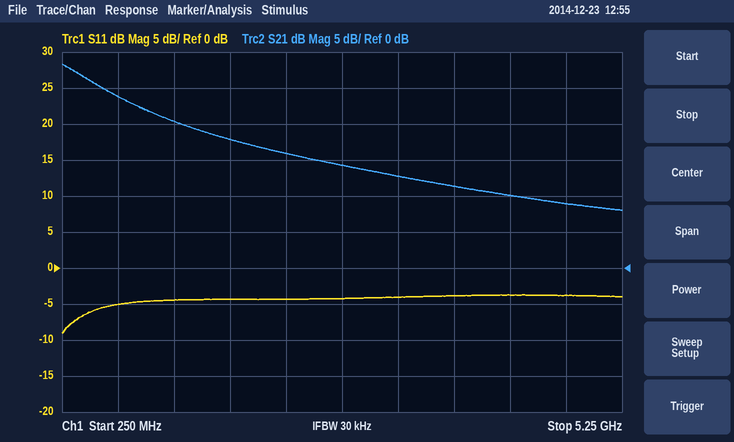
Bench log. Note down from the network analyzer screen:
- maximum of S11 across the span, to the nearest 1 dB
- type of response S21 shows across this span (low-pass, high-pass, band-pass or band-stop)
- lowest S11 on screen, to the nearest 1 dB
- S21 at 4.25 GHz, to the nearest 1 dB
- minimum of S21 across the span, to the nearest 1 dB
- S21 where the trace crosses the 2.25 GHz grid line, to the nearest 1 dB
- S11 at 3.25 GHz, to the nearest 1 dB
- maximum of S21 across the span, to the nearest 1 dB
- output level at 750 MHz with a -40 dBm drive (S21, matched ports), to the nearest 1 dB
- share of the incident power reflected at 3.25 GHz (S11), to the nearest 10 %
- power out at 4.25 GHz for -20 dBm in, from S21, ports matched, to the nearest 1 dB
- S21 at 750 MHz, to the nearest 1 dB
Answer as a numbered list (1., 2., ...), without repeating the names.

1. -4 dB
2. low-pass
3. -9 dB
4. 10 dB
5. 8 dB
6. 16 dB
7. -4 dB
8. 28 dB
9. -16 dBm
10. 40 %
11. -10 dBm
12. 24 dB
